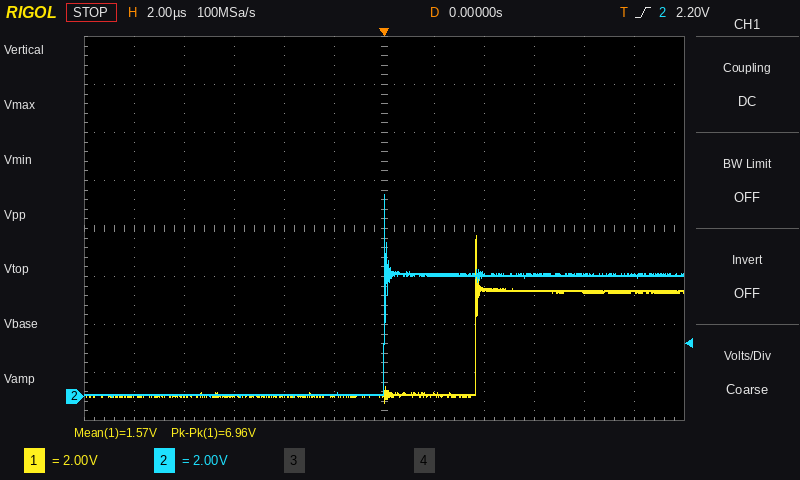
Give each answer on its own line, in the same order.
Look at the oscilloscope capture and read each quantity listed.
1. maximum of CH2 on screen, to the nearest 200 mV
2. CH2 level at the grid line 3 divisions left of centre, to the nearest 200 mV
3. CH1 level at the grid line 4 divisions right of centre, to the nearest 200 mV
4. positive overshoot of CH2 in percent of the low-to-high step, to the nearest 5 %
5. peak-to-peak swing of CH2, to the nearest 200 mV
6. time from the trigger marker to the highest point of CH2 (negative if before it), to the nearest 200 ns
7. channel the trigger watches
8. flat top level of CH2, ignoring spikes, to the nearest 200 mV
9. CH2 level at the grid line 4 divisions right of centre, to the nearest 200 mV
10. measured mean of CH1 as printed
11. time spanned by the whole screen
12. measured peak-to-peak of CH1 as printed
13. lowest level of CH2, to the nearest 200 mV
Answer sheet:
8.4 V
0.0 V
4.4 V
65 %
8.4 V
0.0 µs
CH2
5.0 V
5.0 V
1.57 V
24 µs
6.96 V
0.0 V
